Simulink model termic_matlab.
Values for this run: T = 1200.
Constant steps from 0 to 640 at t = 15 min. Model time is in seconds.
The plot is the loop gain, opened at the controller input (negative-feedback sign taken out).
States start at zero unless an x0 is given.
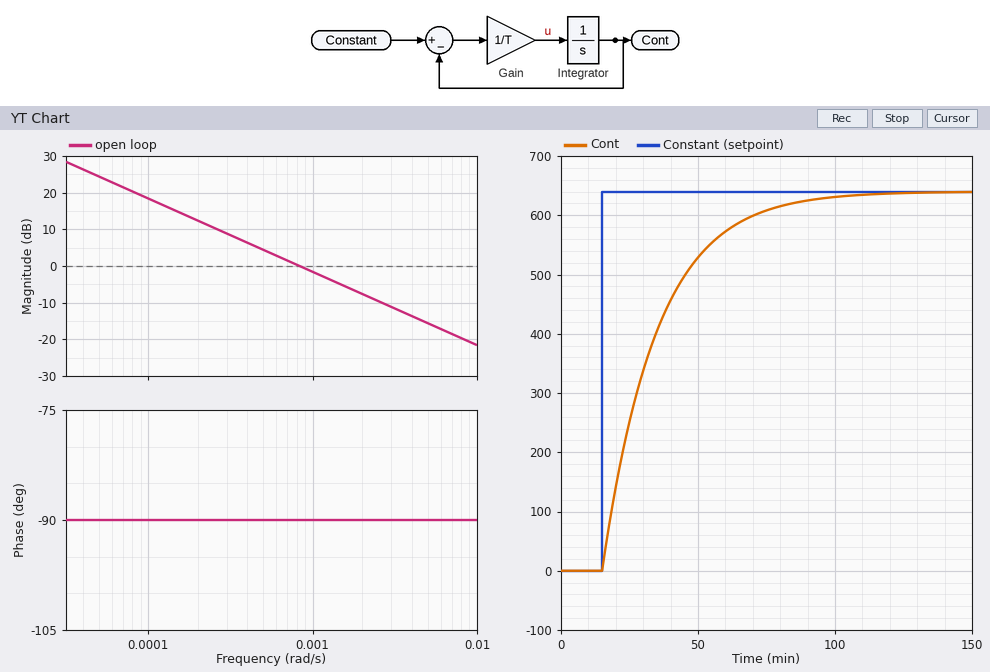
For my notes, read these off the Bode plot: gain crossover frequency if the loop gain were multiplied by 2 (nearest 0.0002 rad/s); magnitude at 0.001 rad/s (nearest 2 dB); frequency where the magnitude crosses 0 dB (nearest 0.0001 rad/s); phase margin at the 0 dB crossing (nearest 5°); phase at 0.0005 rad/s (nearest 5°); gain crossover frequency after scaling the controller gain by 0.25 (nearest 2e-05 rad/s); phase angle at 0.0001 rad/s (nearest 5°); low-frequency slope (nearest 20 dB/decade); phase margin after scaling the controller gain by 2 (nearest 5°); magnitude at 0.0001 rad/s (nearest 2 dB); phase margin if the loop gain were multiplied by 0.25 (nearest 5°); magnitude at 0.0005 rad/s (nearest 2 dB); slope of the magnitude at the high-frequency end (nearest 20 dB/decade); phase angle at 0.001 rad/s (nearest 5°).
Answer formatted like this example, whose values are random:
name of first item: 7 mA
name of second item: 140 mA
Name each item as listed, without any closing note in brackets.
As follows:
gain crossover frequency if the loop gain were multiplied by 2: 0.0016 rad/s
magnitude at 0.001 rad/s: -2 dB
frequency where the magnitude crosses 0 dB: 0.0008 rad/s
phase margin at the 0 dB crossing: 90°
phase at 0.0005 rad/s: -90°
gain crossover frequency after scaling the controller gain by 0.25: 0.00020 rad/s
phase angle at 0.0001 rad/s: -90°
low-frequency slope: -20 dB/decade
phase margin after scaling the controller gain by 2: 90°
magnitude at 0.0001 rad/s: 18 dB
phase margin if the loop gain were multiplied by 0.25: 90°
magnitude at 0.0005 rad/s: 4 dB
slope of the magnitude at the high-frequency end: -20 dB/decade
phase angle at 0.001 rad/s: -90°
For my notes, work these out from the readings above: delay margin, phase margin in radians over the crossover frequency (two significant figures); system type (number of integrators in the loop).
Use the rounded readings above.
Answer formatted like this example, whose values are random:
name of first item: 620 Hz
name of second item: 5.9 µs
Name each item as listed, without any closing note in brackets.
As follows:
delay margin, phase margin in radians over the crossover frequency: 2000 s
system type: 1
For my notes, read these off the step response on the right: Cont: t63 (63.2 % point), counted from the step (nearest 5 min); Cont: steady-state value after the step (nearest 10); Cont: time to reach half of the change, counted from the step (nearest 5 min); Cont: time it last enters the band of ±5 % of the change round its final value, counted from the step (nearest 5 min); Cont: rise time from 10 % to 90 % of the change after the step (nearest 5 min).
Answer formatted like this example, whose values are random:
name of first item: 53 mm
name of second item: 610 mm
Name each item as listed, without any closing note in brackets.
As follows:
Cont: t63 (63.2 % point), counted from the step: 20 min
Cont: steady-state value after the step: 640
Cont: time to reach half of the change, counted from the step: 15 min
Cont: time it last enters the band of ±5 % of the change round its final value, counted from the step: 60 min
Cont: rise time from 10 % to 90 % of the change after the step: 45 min
